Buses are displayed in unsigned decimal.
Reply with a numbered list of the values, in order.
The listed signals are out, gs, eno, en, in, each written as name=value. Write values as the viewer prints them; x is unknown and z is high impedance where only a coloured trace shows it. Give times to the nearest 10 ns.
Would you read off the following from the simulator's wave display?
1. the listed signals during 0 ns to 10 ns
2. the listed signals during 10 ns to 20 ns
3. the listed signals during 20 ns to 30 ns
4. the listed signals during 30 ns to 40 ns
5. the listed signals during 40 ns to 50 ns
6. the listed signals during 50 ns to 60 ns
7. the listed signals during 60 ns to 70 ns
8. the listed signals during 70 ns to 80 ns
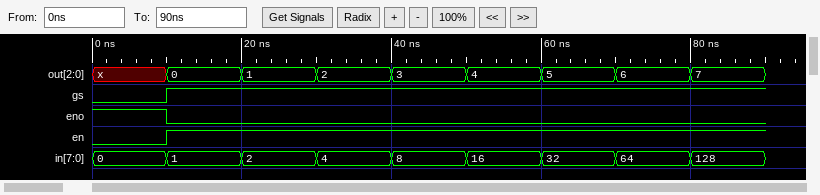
1. out=x, gs=0, eno=1, en=0, in=0
2. out=0, gs=1, eno=0, en=1, in=1
3. out=1, gs=1, eno=0, en=1, in=2
4. out=2, gs=1, eno=0, en=1, in=4
5. out=3, gs=1, eno=0, en=1, in=8
6. out=4, gs=1, eno=0, en=1, in=16
7. out=5, gs=1, eno=0, en=1, in=32
8. out=6, gs=1, eno=0, en=1, in=64
